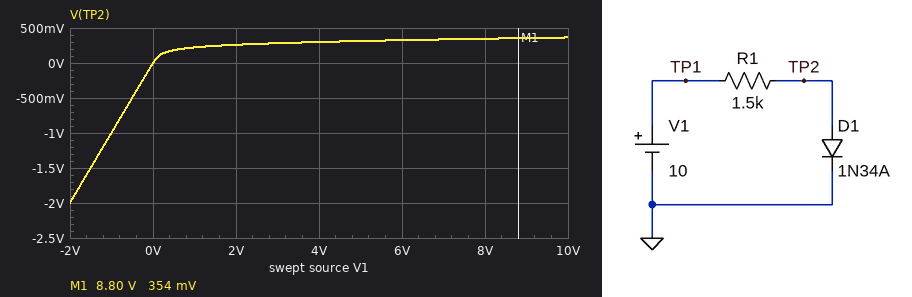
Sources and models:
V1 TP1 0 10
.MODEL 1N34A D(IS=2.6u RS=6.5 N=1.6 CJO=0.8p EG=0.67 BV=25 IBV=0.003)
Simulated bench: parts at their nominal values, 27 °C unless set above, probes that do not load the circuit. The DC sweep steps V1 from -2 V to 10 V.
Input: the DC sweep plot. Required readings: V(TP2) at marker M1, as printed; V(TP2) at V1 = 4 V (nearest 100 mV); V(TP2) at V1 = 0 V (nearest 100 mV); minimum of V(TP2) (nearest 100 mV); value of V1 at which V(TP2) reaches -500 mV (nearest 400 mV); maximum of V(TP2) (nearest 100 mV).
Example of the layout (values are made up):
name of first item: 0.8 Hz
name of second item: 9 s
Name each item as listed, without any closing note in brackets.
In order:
V(TP2) at marker M1, as printed: 354 mV
V(TP2) at V1 = 4 V: 300 mV
V(TP2) at V1 = 0 V: 0 V
minimum of V(TP2): -2.0 V
value of V1 at which V(TP2) reaches -500 mV: -400 mV
maximum of V(TP2): 400 mV
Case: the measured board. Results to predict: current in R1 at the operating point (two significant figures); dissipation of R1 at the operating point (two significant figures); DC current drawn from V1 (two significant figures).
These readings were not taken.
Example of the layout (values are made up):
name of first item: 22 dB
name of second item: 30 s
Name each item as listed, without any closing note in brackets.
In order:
current in R1 at the operating point: 6.4 mA
dissipation of R1 at the operating point: 62 mW
DC current drawn from V1: 6.4 mA
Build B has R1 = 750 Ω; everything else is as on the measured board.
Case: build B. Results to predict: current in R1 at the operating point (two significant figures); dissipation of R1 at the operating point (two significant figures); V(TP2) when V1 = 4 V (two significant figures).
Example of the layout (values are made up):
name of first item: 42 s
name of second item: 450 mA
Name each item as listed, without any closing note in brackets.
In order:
current in R1 at the operating point: 13 mA
dissipation of R1 at the operating point: 120 mW
V(TP2) when V1 = 4 V: 340 mV
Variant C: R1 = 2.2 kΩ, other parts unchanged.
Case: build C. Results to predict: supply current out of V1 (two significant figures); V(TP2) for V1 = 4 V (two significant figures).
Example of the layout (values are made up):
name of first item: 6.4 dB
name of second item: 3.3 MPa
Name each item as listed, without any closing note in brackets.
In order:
supply current out of V1: 4.4 mA
V(TP2) for V1 = 4 V: 280 mV
